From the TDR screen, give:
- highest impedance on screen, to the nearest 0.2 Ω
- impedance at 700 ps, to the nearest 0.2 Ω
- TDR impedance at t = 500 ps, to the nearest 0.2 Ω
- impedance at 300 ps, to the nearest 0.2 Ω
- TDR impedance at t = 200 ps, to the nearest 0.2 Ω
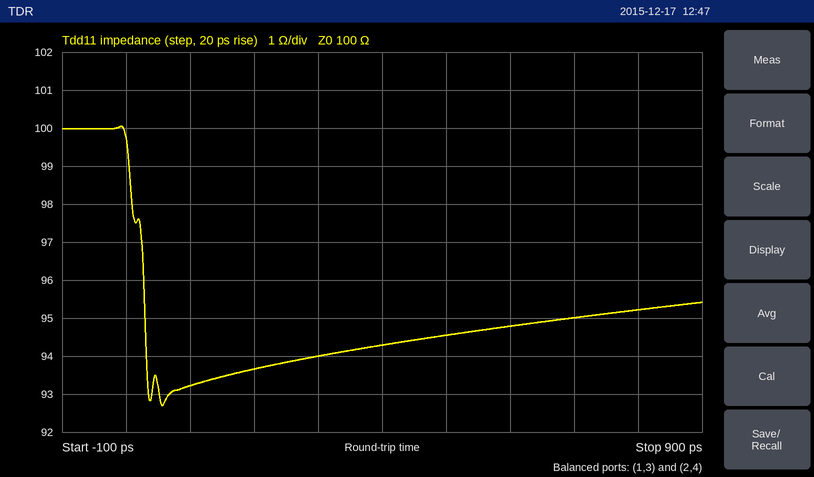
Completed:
100.0 Ω
95.0 Ω
94.6 Ω
94.0 Ω
93.6 Ω
